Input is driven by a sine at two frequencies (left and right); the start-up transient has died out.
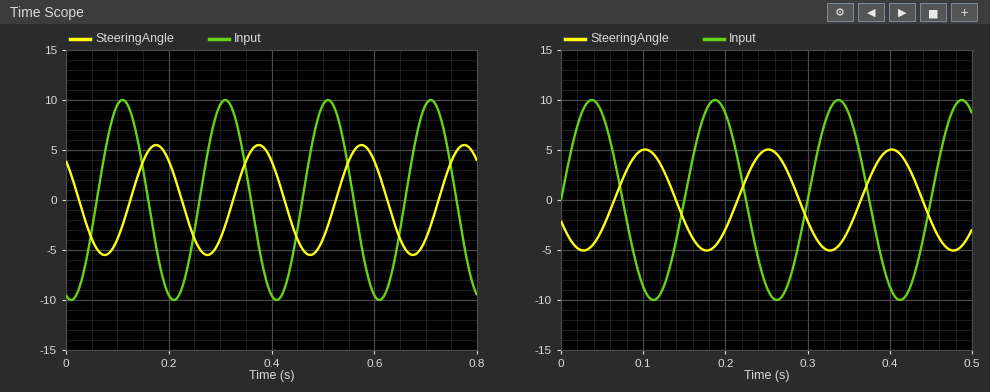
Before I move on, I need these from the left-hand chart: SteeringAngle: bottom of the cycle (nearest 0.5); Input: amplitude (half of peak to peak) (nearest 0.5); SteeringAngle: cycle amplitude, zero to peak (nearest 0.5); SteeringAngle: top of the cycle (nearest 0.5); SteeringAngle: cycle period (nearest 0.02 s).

-5.5
10.0
5.5
5.5
0.20 s
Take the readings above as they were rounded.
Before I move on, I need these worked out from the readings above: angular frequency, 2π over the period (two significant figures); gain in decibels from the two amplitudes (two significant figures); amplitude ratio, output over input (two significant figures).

31 rad/s
-5.2 dB
0.55
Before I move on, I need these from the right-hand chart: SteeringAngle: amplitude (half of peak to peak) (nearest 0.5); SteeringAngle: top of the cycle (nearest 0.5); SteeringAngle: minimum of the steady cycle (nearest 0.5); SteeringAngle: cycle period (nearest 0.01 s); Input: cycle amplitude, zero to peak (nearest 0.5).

5.0
5.0
-5.0
0.15 s
10.0
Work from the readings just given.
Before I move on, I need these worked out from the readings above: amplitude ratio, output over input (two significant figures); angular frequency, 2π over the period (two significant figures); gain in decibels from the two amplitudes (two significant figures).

0.50
42 rad/s
-6.0 dB
